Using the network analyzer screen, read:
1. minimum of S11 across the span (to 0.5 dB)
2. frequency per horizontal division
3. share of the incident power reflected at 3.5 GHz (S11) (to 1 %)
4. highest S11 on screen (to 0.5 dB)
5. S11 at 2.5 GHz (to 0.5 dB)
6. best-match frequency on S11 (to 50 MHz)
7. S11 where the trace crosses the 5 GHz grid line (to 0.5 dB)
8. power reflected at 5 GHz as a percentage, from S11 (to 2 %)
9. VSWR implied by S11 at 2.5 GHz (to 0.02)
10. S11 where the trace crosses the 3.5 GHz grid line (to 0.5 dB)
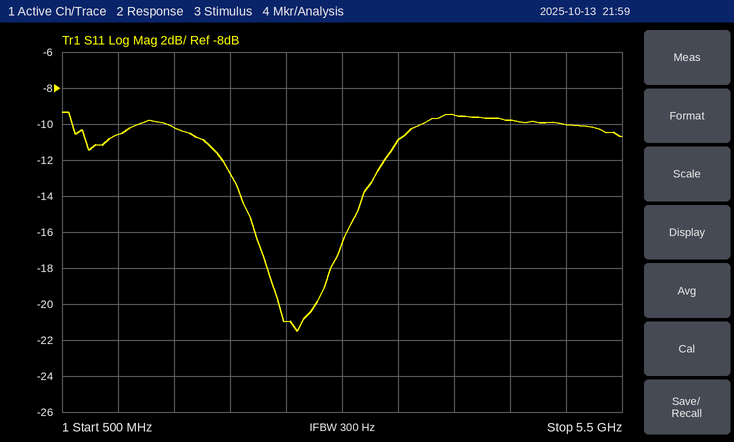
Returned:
-21.5 dB
500 MHz
8 %
-9.5 dB
-21.0 dB
2.60 GHz
-10.0 dB
10 %
1.20
-11.0 dB
